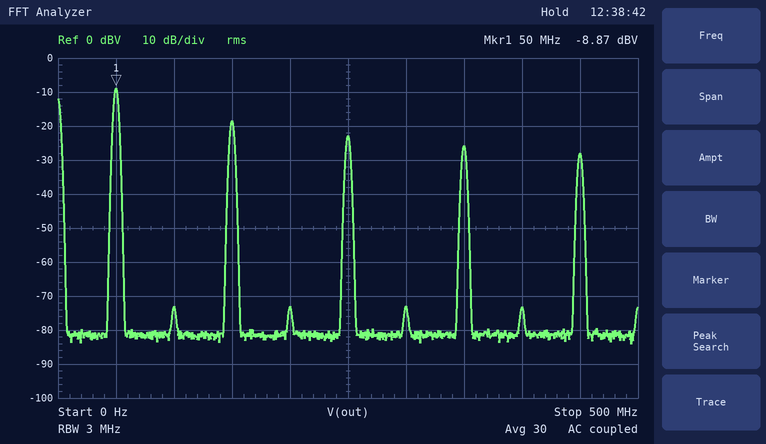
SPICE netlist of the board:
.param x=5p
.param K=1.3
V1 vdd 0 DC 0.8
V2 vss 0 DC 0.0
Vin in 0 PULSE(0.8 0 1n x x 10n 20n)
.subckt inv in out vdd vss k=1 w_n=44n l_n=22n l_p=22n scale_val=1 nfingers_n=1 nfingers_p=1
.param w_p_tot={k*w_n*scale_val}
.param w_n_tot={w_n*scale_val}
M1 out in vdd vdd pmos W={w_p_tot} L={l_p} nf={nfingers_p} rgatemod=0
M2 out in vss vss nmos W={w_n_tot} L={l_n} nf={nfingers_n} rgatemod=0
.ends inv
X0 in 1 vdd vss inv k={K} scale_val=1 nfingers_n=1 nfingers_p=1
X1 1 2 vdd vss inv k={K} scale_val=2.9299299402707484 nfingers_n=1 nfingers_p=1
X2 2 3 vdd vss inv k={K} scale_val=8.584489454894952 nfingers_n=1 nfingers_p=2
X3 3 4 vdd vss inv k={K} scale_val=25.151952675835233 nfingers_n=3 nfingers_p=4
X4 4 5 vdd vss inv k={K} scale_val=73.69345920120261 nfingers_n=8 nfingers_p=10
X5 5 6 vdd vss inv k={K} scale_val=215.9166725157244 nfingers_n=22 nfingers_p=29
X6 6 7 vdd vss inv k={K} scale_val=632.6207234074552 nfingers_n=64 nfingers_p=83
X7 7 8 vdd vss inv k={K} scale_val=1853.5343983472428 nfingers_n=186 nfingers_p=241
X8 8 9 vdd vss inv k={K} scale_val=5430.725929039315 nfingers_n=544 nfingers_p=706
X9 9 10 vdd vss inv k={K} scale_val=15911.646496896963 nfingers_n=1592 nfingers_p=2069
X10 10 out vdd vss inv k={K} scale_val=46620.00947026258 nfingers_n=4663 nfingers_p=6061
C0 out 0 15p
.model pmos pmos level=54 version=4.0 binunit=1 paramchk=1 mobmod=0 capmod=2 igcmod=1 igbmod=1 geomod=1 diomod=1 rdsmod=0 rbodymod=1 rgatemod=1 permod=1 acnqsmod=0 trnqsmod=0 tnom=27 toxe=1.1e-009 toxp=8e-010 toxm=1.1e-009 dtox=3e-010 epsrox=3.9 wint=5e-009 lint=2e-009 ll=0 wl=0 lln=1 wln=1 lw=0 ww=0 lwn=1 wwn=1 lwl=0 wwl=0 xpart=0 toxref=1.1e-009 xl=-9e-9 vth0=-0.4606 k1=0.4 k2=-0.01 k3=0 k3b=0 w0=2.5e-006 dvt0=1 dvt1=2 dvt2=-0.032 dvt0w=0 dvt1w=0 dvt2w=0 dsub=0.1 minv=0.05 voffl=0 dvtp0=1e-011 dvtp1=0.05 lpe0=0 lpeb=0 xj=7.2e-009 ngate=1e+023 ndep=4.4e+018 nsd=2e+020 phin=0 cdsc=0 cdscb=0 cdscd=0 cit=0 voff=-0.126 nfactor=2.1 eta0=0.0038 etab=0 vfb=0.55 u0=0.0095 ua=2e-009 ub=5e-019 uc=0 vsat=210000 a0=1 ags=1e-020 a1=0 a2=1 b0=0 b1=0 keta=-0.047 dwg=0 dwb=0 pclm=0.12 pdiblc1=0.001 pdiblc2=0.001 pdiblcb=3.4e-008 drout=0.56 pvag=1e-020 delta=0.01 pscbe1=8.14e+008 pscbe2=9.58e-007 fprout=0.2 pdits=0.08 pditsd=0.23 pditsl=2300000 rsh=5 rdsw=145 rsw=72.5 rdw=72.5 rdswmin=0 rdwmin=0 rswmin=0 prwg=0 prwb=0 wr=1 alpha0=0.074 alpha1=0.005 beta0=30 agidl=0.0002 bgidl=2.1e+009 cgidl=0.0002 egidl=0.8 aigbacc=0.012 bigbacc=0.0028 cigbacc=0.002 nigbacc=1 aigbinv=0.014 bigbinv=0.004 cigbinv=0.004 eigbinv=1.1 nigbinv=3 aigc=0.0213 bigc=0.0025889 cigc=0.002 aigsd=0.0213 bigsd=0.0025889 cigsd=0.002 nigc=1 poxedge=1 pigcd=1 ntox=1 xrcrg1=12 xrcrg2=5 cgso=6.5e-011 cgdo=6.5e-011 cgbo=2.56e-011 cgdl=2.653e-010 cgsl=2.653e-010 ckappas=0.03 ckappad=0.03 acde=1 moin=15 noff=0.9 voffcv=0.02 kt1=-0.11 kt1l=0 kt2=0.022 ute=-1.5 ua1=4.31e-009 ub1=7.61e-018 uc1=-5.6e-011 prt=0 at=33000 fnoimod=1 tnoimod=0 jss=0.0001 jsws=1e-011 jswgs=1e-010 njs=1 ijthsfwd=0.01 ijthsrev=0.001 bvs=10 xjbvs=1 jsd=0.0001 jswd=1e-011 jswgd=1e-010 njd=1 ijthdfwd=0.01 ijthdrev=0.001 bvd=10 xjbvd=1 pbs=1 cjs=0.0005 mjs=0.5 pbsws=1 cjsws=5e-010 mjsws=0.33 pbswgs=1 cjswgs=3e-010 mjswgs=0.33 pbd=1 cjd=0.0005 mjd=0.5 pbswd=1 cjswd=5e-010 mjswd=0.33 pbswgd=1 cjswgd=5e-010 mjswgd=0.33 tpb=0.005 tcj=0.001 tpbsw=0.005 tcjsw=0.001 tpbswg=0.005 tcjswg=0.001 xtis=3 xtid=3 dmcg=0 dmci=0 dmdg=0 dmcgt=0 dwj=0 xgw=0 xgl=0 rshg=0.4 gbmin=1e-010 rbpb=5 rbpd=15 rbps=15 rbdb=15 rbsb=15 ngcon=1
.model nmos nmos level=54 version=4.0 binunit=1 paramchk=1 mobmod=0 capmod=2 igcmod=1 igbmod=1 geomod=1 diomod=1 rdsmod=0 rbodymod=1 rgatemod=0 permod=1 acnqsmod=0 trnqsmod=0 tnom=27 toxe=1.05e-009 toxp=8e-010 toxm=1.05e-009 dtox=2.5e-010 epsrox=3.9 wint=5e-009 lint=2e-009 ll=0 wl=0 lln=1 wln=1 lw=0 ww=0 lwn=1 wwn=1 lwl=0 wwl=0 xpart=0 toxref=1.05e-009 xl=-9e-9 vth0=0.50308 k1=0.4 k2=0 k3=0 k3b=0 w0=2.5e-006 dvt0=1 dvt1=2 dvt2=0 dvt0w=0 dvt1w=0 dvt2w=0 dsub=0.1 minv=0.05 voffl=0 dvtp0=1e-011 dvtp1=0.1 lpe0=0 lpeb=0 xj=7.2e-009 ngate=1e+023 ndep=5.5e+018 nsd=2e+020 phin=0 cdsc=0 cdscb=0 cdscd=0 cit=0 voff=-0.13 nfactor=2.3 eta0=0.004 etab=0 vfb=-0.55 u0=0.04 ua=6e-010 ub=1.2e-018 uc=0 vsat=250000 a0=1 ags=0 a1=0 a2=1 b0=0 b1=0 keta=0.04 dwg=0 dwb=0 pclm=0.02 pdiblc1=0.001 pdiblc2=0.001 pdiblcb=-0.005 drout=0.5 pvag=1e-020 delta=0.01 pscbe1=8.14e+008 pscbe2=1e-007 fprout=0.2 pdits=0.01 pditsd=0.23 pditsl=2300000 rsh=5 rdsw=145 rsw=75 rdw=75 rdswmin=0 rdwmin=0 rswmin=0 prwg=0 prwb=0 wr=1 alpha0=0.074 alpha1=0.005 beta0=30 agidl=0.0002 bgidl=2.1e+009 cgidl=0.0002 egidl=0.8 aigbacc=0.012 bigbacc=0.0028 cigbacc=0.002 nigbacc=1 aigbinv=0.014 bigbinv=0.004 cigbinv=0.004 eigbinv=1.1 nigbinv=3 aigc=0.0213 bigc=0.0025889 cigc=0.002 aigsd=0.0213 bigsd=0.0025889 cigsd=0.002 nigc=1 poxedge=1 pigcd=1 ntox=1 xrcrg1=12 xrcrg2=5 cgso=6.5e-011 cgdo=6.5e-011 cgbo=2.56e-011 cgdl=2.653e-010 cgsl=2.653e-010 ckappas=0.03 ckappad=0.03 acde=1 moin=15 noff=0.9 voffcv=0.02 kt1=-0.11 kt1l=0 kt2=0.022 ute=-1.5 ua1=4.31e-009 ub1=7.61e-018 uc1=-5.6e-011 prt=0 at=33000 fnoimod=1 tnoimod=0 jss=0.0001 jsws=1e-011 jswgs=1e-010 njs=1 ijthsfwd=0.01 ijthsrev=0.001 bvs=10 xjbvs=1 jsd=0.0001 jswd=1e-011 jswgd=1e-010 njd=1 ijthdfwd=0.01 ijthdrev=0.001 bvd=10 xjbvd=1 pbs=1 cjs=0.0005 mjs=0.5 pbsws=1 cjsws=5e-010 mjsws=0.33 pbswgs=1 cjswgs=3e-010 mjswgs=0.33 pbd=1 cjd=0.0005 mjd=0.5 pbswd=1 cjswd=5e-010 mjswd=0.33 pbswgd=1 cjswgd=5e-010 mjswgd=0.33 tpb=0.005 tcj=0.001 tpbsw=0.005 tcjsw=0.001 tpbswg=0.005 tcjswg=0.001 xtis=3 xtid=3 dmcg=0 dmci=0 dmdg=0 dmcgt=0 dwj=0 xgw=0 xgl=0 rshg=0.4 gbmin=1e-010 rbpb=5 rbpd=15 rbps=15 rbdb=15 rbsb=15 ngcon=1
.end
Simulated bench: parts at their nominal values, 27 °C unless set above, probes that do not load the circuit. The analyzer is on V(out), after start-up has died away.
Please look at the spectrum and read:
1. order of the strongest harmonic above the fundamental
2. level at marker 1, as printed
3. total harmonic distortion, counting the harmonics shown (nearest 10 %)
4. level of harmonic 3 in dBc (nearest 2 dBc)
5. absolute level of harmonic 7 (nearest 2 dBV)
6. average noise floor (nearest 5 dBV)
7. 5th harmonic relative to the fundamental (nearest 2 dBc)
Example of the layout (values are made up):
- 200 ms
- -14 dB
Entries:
- 3
- -8.87 dBV
- 40 %
- -10 dBc
- -26 dBV
- -80 dBV
- -14 dBc
